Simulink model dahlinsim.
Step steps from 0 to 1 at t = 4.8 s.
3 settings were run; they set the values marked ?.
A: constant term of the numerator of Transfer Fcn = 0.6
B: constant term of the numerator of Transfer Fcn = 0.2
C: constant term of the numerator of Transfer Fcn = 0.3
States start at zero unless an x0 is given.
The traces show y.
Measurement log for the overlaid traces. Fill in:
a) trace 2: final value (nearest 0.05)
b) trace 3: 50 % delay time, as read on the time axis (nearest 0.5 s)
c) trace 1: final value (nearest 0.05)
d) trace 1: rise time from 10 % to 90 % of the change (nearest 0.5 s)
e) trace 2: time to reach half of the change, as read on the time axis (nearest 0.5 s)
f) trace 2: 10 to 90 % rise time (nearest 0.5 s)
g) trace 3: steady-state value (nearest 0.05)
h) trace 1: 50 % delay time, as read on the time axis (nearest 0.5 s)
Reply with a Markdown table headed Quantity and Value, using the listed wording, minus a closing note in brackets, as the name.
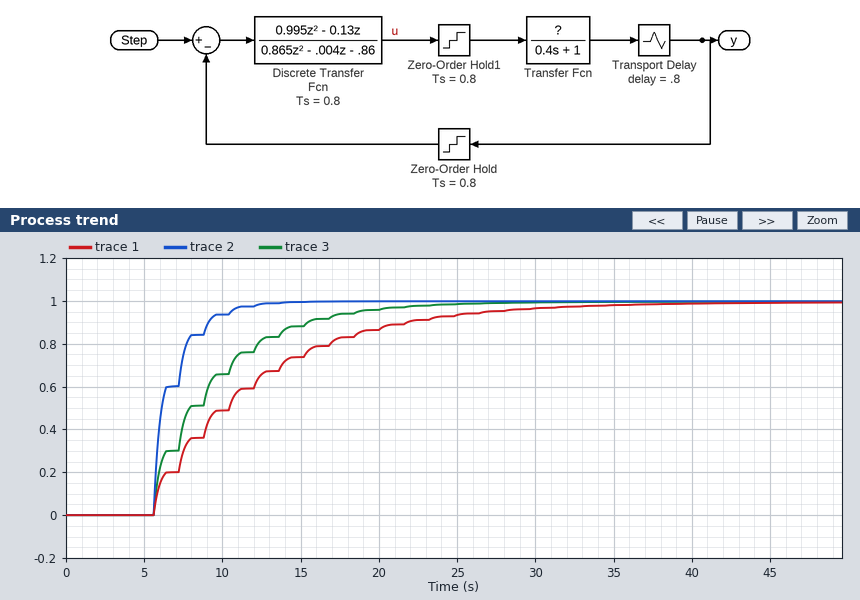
| Quantity | Value |
|---|---|
| trace 2: final value | 1.00 |
| trace 3: 50 % delay time, as read on the time axis | 8.0 s |
| trace 1: final value | 1.00 |
| trace 1: rise time from 10 % to 90 % of the change | 16.0 s |
| trace 2: time to reach half of the change, as read on the time axis | 6.0 s |
| trace 2: 10 to 90 % rise time | 3.5 s |
| trace 3: steady-state value | 1.00 |
| trace 1: 50 % delay time, as read on the time axis | 10.5 s |
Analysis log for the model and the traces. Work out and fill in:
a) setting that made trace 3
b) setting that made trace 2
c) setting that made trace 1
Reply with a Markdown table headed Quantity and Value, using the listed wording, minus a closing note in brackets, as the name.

| Quantity | Value |
|---|---|
| setting that made trace 3 | C |
| setting that made trace 2 | A |
| setting that made trace 1 | B |
